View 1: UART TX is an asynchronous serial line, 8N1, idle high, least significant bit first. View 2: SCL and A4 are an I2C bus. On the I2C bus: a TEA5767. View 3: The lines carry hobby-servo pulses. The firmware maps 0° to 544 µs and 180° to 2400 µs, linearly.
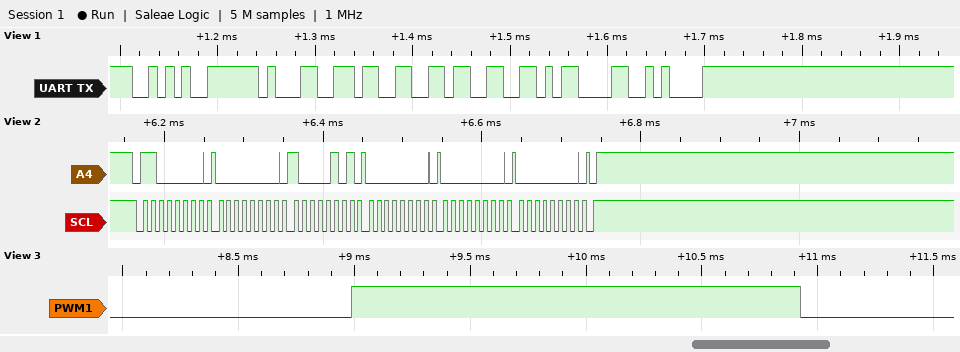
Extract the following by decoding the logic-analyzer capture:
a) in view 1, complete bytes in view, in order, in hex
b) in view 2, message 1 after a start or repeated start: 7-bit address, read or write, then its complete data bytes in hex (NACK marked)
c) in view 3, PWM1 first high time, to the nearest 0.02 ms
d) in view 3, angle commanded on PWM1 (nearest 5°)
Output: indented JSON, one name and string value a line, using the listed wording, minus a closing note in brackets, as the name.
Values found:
{
  "in view 1, complete bytes in view, in order, in hex": "2A 31 33 33 0D 0A",
  "in view 2, message 1 after a start or repeated start: 7-bit address, read or write, then its complete data bytes in hex": "0x60 write: 00 85 00 00 00",
  "in view 3, PWM1 first high time, to the nearest 0.02 ms": "1.94 ms",
  "in view 3, angle commanded on PWM1": "135°"
}
